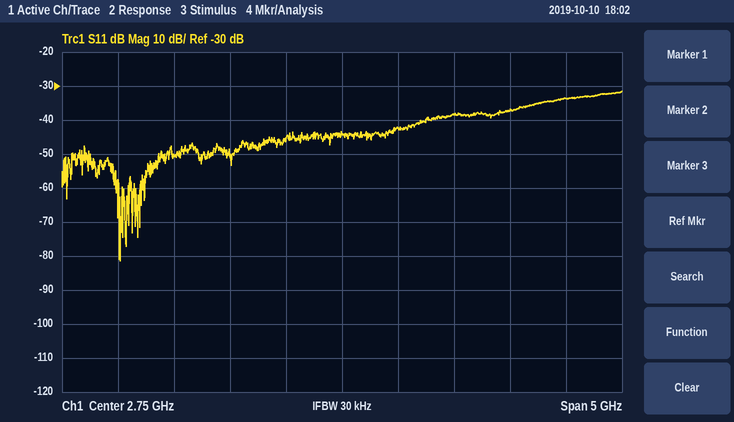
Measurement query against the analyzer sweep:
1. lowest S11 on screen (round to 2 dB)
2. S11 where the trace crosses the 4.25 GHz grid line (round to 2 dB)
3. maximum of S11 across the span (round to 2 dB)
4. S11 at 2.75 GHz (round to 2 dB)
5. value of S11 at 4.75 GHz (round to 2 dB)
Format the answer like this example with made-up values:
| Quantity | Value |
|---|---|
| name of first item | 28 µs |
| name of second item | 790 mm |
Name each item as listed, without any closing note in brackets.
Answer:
| Quantity | Value |
|---|---|
| lowest S11 on screen | -82 dB |
| S11 where the trace crosses the 4.25 GHz grid line | -38 dB |
| maximum of S11 across the span | -32 dB |
| S11 at 2.75 GHz | -44 dB |
| value of S11 at 4.75 GHz | -34 dB |
